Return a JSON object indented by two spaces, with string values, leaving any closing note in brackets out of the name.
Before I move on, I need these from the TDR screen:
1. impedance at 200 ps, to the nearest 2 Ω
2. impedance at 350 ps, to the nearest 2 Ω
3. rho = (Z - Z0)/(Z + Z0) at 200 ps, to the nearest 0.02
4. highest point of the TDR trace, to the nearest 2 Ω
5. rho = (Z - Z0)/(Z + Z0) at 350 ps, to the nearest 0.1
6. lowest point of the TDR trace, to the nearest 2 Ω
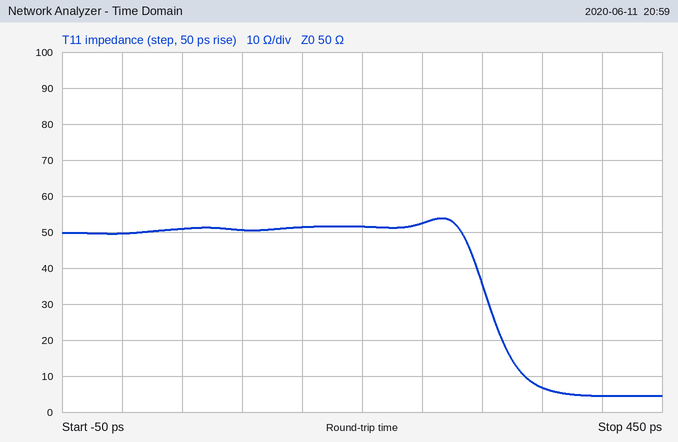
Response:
{
  "impedance at 200 ps, to the nearest 2 Ω": "52 Ω",
  "impedance at 350 ps, to the nearest 2 Ω": "6 Ω",
  "rho = (Z - Z0)/(Z + Z0) at 200 ps, to the nearest 0.02": "+0.02",
  "highest point of the TDR trace, to the nearest 2 Ω": "54 Ω",
  "rho = (Z - Z0)/(Z + Z0) at 350 ps, to the nearest 0.1": "-0.8",
  "lowest point of the TDR trace, to the nearest 2 Ω": "4 Ω"
}
